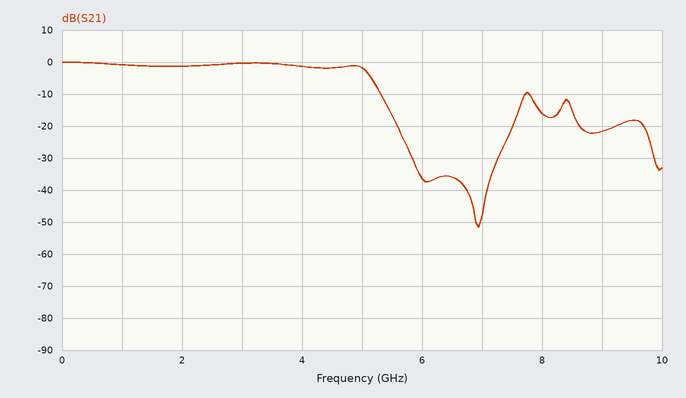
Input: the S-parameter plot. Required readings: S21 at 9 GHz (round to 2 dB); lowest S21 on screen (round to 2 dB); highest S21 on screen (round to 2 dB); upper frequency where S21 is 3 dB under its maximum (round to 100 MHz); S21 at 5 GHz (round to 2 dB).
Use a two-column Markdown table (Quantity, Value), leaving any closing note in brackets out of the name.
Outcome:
| Quantity | Value |
|---|---|
| S21 at 9 GHz | -22 dB |
| lowest S21 on screen | -52 dB |
| highest S21 on screen | 0 dB |
| upper frequency where S21 is 3 dB under its maximum | 5.1 GHz |
| S21 at 5 GHz | -2 dB |
